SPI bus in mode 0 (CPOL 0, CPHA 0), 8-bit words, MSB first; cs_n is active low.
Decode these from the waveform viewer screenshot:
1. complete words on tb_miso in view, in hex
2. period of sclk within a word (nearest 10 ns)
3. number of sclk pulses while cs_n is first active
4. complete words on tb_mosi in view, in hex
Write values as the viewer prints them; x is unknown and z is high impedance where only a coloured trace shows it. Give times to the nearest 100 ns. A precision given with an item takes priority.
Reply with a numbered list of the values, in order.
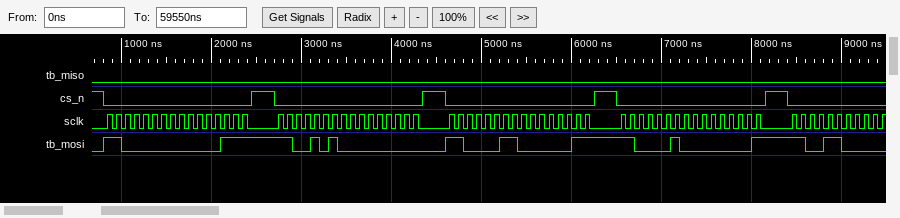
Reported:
1. 00, 00, 00, 00, 00, 00, 00, 00, 00
2. 100 ns
3. 16
4. C0, 07, CA, 00, C3, 03, C2, 01, CC
